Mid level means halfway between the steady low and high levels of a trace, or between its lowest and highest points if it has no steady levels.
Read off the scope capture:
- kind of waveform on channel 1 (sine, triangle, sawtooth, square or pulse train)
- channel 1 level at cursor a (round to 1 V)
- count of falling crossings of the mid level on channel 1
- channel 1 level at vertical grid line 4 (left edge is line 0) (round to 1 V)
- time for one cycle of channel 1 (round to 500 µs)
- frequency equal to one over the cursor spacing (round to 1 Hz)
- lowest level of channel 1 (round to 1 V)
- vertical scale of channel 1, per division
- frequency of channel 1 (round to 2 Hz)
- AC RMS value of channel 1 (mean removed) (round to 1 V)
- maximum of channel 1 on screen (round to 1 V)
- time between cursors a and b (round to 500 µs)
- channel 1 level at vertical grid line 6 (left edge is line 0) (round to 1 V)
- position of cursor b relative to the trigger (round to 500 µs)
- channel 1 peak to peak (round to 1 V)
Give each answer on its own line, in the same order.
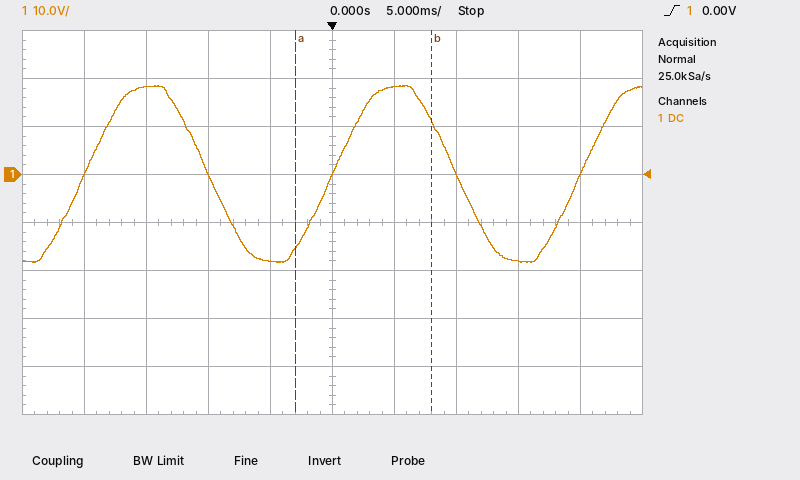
sine
-15 V
2
-18 V
20.0 ms
91 Hz
-18 V
10 V
50 Hz
13 V
19 V
11.0 ms
18 V
+8.0 ms
37 V
